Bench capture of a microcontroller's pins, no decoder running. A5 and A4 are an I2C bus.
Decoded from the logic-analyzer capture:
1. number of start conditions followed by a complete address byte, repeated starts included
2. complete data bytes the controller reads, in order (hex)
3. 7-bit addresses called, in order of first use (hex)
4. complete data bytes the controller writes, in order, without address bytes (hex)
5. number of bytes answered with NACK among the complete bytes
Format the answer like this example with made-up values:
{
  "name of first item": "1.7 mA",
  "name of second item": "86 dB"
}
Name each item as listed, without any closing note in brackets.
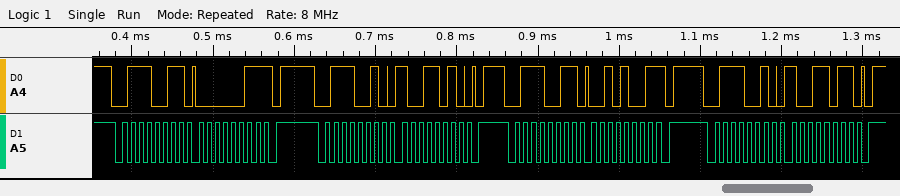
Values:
{
  "number of start conditions followed by a complete address byte, repeated starts included": "4",
  "complete data bytes the controller reads, in order": "03 29",
  "7-bit addresses called, in order of first use": "0x39",
  "complete data bytes the controller writes, in order, without address bytes": "9A 9B",
  "number of bytes answered with NACK among the complete bytes": "2"
}
